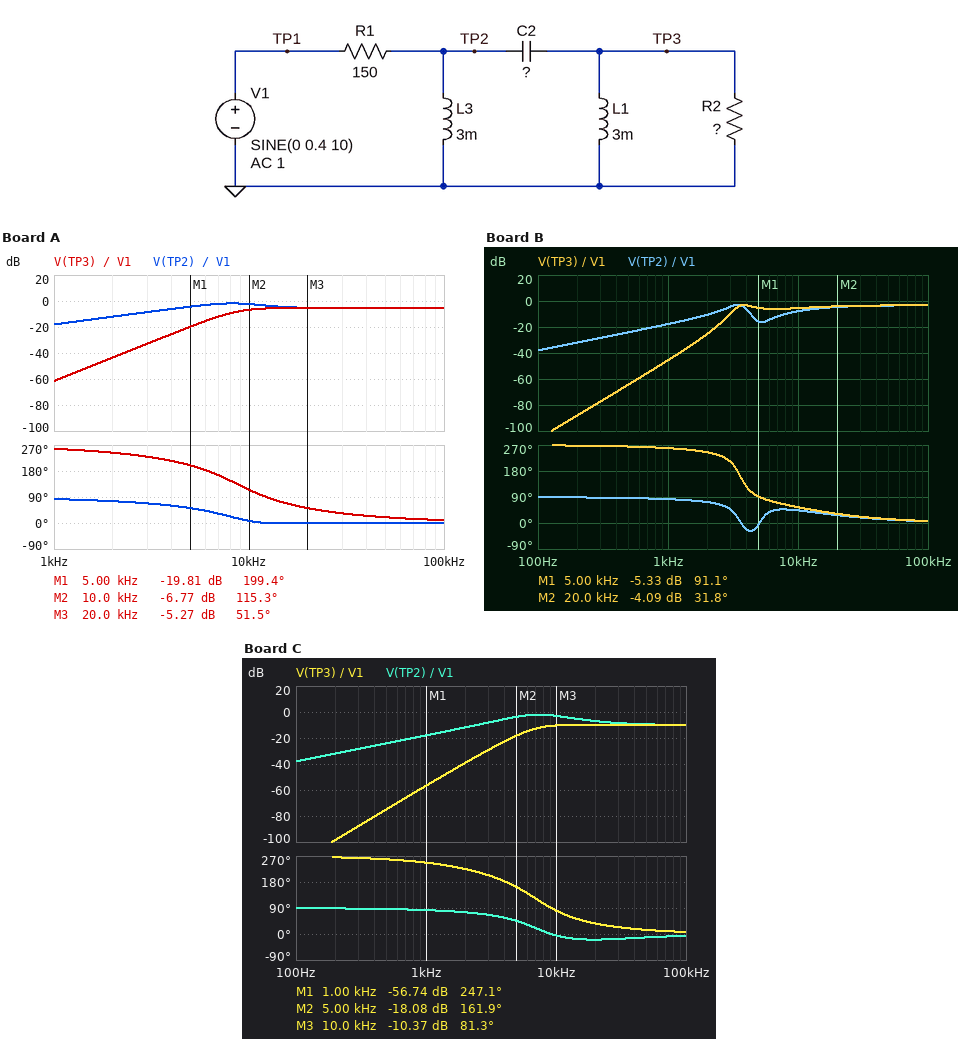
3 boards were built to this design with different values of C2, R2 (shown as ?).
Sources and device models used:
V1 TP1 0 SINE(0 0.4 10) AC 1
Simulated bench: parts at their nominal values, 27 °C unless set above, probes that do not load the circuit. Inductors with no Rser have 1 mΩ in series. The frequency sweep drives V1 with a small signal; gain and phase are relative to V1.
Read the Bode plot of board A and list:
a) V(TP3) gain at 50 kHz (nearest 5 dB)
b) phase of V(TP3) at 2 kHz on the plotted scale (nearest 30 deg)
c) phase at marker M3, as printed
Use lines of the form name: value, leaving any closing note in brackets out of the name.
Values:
V(TP3) gain at 50 kHz: -5 dB
phase of V(TP3) at 2 kHz on the plotted scale: 240 deg
phase at marker M3, as printed: 51.5 deg
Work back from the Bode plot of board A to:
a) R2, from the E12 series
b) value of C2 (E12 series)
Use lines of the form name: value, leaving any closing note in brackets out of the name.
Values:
R2, from the E12 series: 180 Ω
value of C2: 56 nF
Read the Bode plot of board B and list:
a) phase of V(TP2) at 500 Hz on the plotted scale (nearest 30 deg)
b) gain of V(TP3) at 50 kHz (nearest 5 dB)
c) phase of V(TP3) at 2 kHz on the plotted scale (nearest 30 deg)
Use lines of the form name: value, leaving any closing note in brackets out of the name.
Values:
phase of V(TP2) at 500 Hz on the plotted scale: 90 deg
gain of V(TP3) at 50 kHz: -5 dB
phase of V(TP3) at 2 kHz on the plotted scale: 240 deg
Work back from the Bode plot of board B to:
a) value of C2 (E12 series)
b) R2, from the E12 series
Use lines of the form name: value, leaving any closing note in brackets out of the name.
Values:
value of C2: 330 nF
R2, from the E12 series: 330 Ω
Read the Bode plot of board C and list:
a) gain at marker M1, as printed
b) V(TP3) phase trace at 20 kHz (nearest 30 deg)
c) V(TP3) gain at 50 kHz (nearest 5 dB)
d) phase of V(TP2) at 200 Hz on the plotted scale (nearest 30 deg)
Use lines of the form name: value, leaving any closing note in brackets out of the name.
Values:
gain at marker M1, as printed: -56.74 dB
V(TP3) phase trace at 20 kHz: 30 deg
V(TP3) gain at 50 kHz: -10 dB
phase of V(TP2) at 200 Hz on the plotted scale: 90 deg
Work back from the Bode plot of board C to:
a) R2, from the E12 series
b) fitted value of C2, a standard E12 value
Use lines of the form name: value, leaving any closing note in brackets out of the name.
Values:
R2, from the E12 series: 68 Ω
fitted value of C2, a standard E12 value: 100 nF
